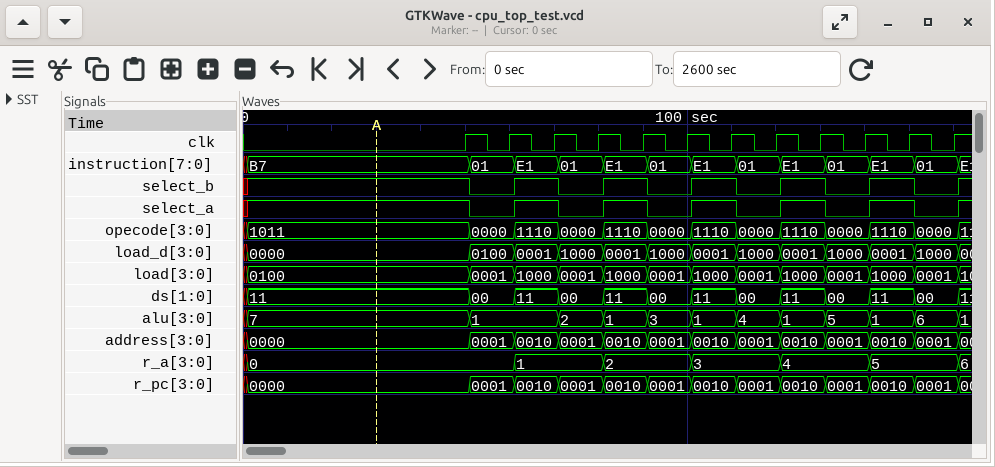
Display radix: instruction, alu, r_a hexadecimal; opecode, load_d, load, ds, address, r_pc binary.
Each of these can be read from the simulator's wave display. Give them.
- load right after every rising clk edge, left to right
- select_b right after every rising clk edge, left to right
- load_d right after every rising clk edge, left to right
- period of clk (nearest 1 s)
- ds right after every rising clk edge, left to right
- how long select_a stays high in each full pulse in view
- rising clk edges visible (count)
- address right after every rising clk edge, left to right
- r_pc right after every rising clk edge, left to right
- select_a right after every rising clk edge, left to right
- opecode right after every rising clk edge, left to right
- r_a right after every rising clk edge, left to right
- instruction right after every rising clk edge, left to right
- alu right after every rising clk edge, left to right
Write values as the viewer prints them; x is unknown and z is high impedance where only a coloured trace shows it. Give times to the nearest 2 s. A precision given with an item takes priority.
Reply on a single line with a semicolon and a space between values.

0100, 0001, 1000, 0001, 1000, 0001, 1000, 0001, 1000, 0001, 1000, 0001; 1 0 1 0 1 0 1 0 1 0 1 0; 0000, 0100, 0001, 1000, 0001, 1000, 0001, 1000, 0001, 1000, 0001, 1000; 10 s; 11, 00, 11, 00, 11, 00, 11, 00, 11, 00, 11, 00; 10 s, 10 s, 10 s, 10 s, 10 s; 12; 0000, 0001, 0010, 0001, 0010, 0001, 0010, 0001, 0010, 0001, 0010, 0001; 0000, 0001, 0010, 0001, 0010, 0001, 0010, 0001, 0010, 0001, 0010, 0001; 1 0 1 0 1 0 1 0 1 0 1 0; 1011, 0000, 1110, 0000, 1110, 0000, 1110, 0000, 1110, 0000, 1110, 0000; 0, 0, 1, 1, 2, 2, 3, 3, 4, 4, 5, 5; B7, 01, E1, 01, E1, 01, E1, 01, E1, 01, E1, 01; 7, 1, 1, 2, 1, 3, 1, 4, 1, 5, 1, 6
